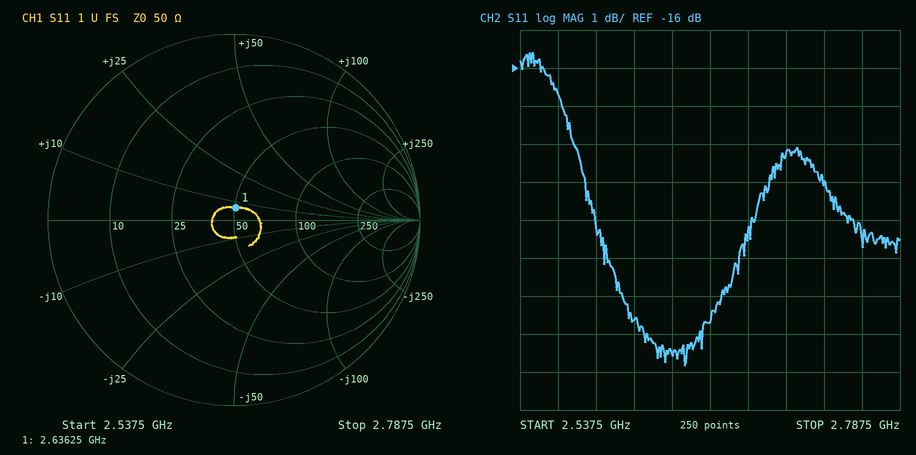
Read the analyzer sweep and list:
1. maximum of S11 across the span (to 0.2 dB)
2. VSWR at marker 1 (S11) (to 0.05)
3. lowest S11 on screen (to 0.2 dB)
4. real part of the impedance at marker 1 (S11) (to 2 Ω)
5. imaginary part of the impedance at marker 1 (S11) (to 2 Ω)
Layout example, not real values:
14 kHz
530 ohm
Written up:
-15.6 dB
1.15
-23.8 dB
50 Ω
+6 Ω
